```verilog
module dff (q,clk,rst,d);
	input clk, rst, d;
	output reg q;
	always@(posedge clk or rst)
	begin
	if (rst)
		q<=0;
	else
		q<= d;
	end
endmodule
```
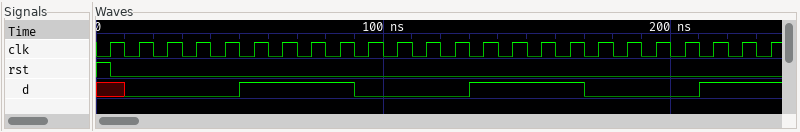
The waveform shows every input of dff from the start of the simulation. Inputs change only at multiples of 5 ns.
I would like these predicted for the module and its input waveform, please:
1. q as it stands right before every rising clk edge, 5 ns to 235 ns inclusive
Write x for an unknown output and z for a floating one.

0 x 0 0 0 0 1 1 1 1 0 0 0 0 1 1 1 1 0 0 0 0 1 1
